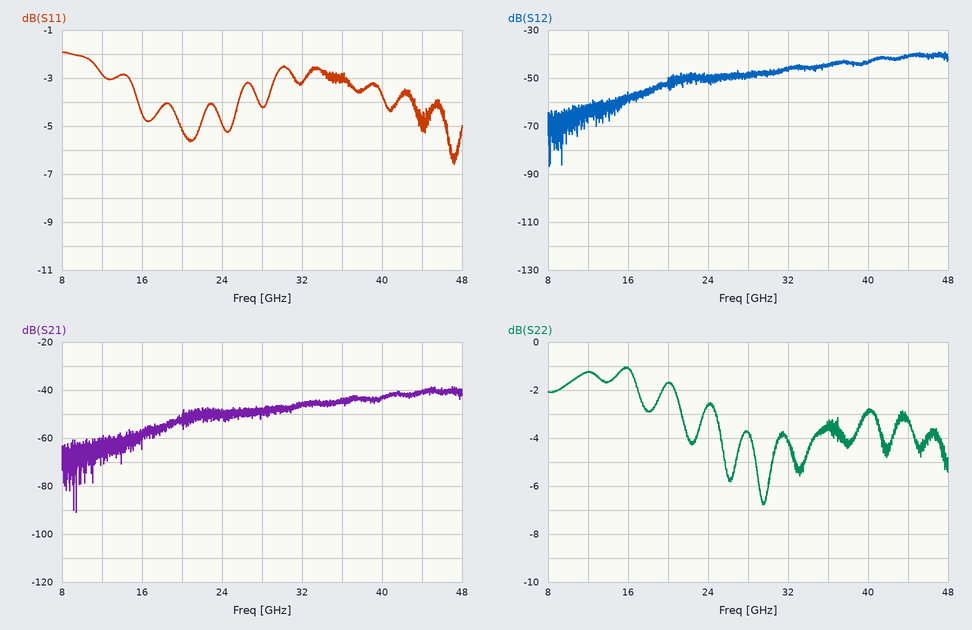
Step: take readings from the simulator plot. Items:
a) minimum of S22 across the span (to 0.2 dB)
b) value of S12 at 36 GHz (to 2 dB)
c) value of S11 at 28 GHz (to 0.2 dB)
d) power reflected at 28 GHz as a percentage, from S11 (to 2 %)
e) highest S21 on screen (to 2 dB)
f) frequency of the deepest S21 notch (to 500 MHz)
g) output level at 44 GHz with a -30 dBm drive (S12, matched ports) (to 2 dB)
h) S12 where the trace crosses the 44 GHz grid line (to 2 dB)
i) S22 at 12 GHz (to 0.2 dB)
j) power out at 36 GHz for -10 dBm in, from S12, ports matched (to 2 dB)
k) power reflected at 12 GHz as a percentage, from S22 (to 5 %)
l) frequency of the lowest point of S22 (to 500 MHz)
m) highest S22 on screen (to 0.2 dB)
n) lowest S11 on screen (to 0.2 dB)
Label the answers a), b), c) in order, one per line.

a) -6.8 dB
b) -44 dB
c) -4.2 dB
d) 38 %
e) -38 dB
f) 9.5 GHz
g) -70 dBm
h) -40 dB
i) -1.2 dB
j) -54 dBm
k) 75 %
l) 29.5 GHz
m) -1.0 dB
n) -6.6 dB
